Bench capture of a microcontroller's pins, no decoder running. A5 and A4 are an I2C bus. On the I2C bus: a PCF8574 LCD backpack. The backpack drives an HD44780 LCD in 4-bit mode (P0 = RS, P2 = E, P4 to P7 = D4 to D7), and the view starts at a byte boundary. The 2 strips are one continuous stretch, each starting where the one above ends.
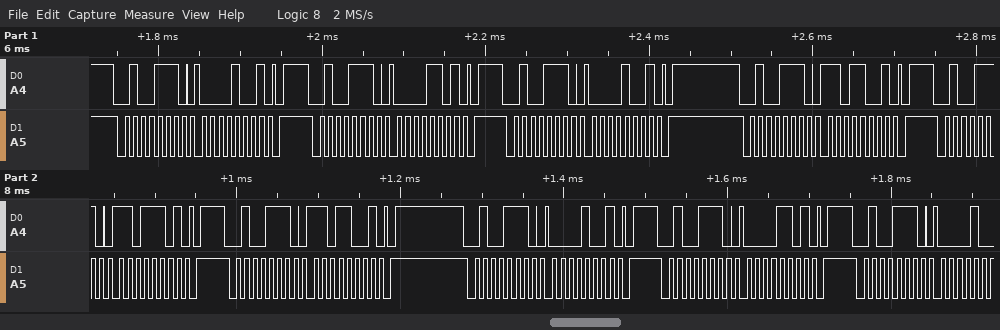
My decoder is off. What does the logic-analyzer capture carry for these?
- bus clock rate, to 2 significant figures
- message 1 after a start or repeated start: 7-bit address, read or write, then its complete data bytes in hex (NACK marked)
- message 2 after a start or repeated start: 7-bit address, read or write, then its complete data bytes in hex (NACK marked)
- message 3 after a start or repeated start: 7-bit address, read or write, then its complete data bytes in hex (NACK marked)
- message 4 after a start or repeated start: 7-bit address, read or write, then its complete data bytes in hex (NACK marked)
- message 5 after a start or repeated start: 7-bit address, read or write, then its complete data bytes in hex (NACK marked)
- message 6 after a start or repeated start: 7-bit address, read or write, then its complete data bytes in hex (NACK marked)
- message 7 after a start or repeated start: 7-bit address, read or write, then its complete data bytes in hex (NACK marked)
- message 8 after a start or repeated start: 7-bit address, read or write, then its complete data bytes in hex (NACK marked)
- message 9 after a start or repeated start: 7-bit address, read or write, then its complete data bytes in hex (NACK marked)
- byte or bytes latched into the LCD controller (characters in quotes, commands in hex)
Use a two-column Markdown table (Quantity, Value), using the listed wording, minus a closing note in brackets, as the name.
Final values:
| Quantity | Value |
|---|---|
| bus clock rate, to 2 significant figures | 100 kHz |
| message 1 after a start or repeated start: 7-bit address, read or write, then its complete data bytes in hex | 0x27 write: 09 |
| message 2 after a start or repeated start: 7-bit address, read or write, then its complete data bytes in hex | 0x27 write: 0D |
| message 3 after a start or repeated start: 7-bit address, read or write, then its complete data bytes in hex | 0x27 write: 09 |
| message 4 after a start or repeated start: 7-bit address, read or write, then its complete data bytes in hex | 0x27 write: D9 |
| message 5 after a start or repeated start: 7-bit address, read or write, then its complete data bytes in hex | 0x27 write: DD |
| message 6 after a start or repeated start: 7-bit address, read or write, then its complete data bytes in hex | 0x27 write: D9 |
| message 7 after a start or repeated start: 7-bit address, read or write, then its complete data bytes in hex | 0x27 write: 09 |
| message 8 after a start or repeated start: 7-bit address, read or write, then its complete data bytes in hex | 0x27 write: 0D |
| message 9 after a start or repeated start: 7-bit address, read or write, then its complete data bytes in hex | 0x27 write |
| byte or bytes latched into the LCD controller | data 0x0D |
